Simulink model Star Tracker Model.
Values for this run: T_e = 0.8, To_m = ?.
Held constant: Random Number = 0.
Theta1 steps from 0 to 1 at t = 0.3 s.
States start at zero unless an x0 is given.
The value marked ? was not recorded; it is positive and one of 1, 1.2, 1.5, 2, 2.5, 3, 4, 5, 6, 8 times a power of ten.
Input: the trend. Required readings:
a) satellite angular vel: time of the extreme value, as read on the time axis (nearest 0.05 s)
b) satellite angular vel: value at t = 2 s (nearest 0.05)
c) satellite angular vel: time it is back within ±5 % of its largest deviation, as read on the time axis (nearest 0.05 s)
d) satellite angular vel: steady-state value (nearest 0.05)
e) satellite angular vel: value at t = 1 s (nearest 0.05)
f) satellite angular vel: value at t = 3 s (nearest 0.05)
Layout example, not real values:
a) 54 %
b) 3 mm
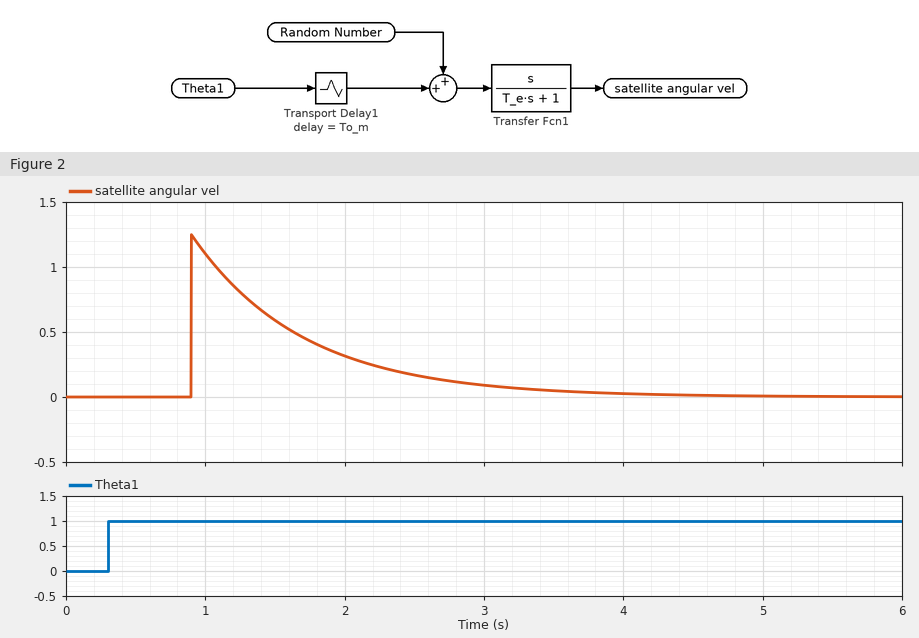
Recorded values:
a) 0.90 s
b) 0.30
c) 3.30 s
d) 0.00
e) 1.10
f) 0.10
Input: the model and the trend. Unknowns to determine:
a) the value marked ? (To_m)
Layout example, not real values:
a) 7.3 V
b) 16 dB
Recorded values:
a) 0.6
